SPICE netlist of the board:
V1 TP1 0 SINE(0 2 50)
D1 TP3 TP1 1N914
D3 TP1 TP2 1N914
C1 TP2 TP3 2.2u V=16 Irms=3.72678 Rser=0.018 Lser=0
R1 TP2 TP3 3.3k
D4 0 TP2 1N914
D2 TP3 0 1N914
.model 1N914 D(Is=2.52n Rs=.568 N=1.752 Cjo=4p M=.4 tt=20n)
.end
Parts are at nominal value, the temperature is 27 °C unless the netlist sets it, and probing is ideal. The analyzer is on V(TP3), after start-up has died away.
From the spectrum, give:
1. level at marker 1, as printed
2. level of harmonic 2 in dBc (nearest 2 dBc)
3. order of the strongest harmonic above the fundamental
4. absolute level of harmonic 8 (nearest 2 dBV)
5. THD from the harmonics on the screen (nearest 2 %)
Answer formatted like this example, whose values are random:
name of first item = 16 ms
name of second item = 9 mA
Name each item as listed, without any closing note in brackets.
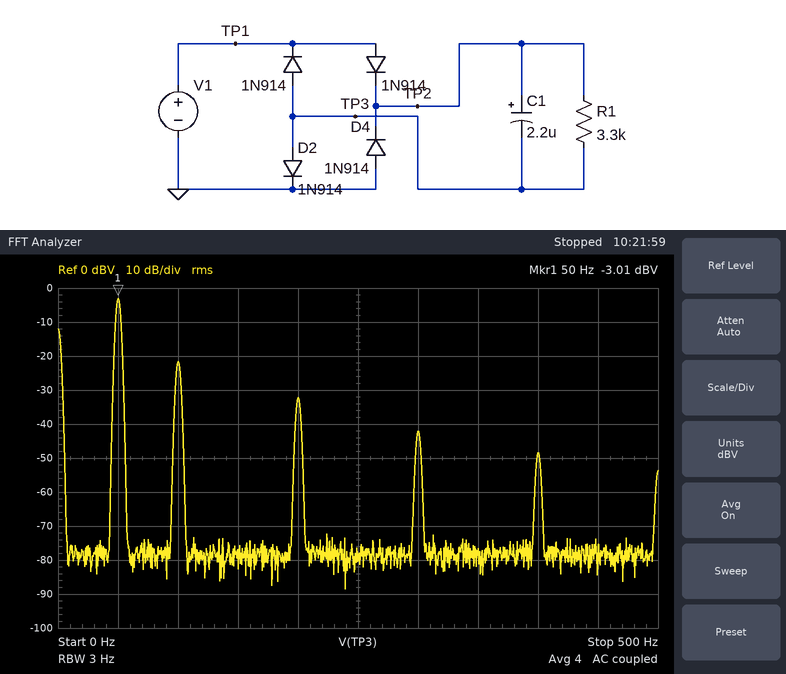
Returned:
level at marker 1, as printed = -3.01 dBV
level of harmonic 2 in dBc = -18 dBc
order of the strongest harmonic above the fundamental = 2
absolute level of harmonic 8 = -48 dBV
THD from the harmonics on the screen = 12 %
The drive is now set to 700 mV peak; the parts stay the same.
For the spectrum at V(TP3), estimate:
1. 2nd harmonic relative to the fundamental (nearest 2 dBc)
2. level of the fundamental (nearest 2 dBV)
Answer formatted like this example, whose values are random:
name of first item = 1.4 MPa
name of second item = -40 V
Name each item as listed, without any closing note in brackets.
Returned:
2nd harmonic relative to the fundamental = -52 dBc
level of the fundamental = -12 dBV
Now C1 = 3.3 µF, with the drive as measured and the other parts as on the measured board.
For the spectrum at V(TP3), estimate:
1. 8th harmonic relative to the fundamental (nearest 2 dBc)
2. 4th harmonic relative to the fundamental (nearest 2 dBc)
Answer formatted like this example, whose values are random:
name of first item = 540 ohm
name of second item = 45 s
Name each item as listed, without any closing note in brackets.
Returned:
8th harmonic relative to the fundamental = -48 dBc
4th harmonic relative to the fundamental = -30 dBc
